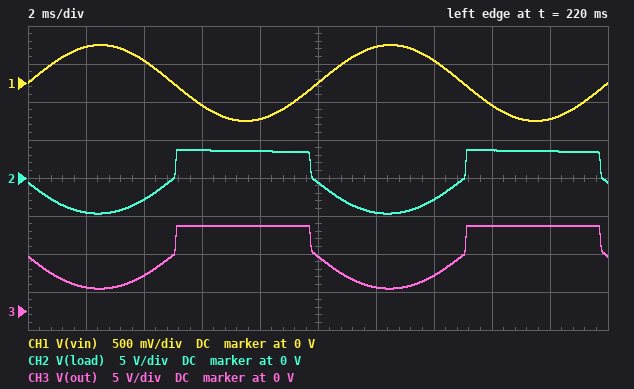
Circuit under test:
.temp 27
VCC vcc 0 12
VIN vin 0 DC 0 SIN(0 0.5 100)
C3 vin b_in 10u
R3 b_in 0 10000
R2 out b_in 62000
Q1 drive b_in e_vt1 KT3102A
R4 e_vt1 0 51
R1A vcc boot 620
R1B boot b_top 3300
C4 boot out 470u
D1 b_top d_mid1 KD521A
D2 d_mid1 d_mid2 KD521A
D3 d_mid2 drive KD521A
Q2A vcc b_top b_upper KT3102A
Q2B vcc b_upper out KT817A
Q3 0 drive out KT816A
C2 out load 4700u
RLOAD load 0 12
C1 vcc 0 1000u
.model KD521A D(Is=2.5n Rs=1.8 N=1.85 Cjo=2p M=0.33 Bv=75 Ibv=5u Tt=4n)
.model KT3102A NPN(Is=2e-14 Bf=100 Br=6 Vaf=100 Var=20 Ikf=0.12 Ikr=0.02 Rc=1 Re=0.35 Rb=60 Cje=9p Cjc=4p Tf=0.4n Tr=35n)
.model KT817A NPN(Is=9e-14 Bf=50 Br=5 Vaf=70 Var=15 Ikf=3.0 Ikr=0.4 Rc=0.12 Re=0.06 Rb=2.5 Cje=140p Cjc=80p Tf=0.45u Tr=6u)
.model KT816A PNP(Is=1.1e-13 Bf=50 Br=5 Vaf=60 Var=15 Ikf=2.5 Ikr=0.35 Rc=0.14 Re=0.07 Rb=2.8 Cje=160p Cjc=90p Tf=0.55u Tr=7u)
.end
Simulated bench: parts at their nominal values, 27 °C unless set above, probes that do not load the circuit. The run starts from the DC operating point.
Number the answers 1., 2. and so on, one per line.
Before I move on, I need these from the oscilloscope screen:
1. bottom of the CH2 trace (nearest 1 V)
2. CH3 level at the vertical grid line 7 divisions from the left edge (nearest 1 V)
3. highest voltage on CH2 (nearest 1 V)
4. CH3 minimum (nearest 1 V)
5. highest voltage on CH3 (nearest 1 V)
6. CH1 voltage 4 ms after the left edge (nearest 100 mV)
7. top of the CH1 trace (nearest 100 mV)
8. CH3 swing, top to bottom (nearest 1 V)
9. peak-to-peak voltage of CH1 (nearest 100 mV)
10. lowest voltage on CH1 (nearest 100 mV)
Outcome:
1. -5 V
2. 5 V
3. 4 V
4. 3 V
5. 11 V
6. 300 mV
7. 500 mV
8. 8 V
9. 1.0 V
10. -500 mV
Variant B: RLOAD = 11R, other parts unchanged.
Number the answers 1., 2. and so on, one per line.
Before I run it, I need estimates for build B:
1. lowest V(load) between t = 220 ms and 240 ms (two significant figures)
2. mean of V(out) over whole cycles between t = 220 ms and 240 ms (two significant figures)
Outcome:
1. -4.4 V
2. 7.8 V
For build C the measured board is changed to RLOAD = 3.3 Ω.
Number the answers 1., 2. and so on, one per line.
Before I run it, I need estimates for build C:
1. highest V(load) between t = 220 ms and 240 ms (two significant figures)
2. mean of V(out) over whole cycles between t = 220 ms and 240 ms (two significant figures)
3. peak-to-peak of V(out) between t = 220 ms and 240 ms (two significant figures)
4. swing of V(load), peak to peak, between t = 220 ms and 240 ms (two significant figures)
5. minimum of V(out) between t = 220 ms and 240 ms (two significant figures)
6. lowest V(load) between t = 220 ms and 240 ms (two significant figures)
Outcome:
1. 2.0 V
2. 9.3 V
3. 3.6 V
4. 3.7 V
5. 7.5 V
6. -1.7 V
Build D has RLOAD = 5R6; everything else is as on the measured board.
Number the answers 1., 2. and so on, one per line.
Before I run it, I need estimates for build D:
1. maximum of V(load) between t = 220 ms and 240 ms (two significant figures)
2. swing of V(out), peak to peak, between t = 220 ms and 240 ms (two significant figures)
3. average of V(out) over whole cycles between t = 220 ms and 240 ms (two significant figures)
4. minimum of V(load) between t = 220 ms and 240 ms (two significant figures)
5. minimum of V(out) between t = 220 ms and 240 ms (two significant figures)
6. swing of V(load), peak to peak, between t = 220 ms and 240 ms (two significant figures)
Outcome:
1. 2.6 V
2. 5.1 V
3. 8.7 V
4. -2.7 V
5. 6.0 V
6. 5.3 V
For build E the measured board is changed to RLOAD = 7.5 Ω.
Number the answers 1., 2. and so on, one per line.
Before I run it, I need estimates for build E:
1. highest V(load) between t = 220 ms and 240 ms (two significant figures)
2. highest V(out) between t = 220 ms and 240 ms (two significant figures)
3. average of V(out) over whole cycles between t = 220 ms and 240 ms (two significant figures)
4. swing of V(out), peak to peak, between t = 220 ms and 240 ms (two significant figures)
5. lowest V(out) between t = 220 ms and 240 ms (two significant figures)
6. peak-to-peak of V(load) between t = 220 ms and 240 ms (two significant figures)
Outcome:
1. 3.0 V
2. 11 V
3. 8.3 V
4. 6.2 V
5. 5.0 V
6. 6.3 V
